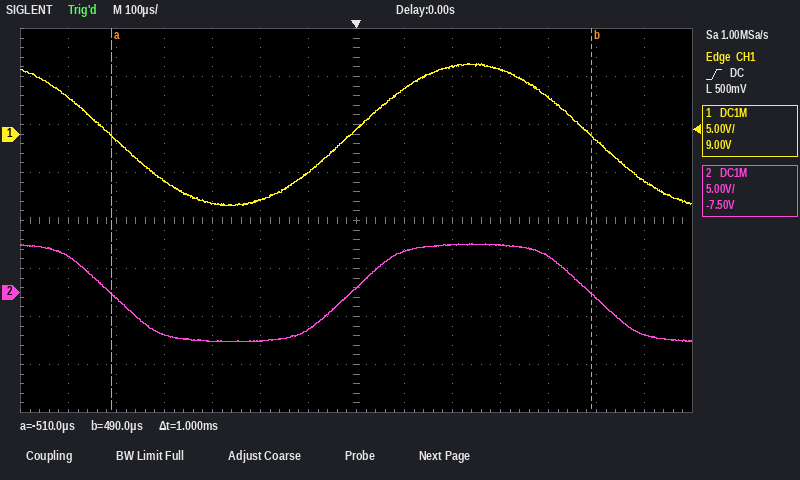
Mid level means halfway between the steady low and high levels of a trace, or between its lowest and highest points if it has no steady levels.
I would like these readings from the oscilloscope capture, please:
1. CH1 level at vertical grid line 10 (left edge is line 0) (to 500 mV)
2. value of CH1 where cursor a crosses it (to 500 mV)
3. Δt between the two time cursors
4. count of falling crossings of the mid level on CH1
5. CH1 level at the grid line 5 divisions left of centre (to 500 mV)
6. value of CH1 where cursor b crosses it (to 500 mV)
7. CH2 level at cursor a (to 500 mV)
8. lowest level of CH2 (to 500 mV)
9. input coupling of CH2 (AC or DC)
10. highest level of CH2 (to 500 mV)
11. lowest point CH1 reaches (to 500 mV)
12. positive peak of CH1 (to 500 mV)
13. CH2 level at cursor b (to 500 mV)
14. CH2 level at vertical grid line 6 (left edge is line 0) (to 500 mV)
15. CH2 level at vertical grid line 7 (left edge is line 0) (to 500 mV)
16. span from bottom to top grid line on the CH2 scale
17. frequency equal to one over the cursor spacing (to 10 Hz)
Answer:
6.5 V
0.0 V
1 ms
2
-500 mV
0.0 V
0.0 V
-5.0 V
DC
5.0 V
-7.5 V
7.5 V
0.0 V
-4.0 V
500 mV
40 V
1.00 kHz
